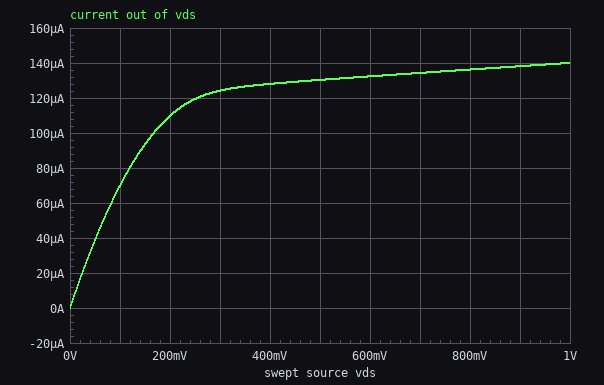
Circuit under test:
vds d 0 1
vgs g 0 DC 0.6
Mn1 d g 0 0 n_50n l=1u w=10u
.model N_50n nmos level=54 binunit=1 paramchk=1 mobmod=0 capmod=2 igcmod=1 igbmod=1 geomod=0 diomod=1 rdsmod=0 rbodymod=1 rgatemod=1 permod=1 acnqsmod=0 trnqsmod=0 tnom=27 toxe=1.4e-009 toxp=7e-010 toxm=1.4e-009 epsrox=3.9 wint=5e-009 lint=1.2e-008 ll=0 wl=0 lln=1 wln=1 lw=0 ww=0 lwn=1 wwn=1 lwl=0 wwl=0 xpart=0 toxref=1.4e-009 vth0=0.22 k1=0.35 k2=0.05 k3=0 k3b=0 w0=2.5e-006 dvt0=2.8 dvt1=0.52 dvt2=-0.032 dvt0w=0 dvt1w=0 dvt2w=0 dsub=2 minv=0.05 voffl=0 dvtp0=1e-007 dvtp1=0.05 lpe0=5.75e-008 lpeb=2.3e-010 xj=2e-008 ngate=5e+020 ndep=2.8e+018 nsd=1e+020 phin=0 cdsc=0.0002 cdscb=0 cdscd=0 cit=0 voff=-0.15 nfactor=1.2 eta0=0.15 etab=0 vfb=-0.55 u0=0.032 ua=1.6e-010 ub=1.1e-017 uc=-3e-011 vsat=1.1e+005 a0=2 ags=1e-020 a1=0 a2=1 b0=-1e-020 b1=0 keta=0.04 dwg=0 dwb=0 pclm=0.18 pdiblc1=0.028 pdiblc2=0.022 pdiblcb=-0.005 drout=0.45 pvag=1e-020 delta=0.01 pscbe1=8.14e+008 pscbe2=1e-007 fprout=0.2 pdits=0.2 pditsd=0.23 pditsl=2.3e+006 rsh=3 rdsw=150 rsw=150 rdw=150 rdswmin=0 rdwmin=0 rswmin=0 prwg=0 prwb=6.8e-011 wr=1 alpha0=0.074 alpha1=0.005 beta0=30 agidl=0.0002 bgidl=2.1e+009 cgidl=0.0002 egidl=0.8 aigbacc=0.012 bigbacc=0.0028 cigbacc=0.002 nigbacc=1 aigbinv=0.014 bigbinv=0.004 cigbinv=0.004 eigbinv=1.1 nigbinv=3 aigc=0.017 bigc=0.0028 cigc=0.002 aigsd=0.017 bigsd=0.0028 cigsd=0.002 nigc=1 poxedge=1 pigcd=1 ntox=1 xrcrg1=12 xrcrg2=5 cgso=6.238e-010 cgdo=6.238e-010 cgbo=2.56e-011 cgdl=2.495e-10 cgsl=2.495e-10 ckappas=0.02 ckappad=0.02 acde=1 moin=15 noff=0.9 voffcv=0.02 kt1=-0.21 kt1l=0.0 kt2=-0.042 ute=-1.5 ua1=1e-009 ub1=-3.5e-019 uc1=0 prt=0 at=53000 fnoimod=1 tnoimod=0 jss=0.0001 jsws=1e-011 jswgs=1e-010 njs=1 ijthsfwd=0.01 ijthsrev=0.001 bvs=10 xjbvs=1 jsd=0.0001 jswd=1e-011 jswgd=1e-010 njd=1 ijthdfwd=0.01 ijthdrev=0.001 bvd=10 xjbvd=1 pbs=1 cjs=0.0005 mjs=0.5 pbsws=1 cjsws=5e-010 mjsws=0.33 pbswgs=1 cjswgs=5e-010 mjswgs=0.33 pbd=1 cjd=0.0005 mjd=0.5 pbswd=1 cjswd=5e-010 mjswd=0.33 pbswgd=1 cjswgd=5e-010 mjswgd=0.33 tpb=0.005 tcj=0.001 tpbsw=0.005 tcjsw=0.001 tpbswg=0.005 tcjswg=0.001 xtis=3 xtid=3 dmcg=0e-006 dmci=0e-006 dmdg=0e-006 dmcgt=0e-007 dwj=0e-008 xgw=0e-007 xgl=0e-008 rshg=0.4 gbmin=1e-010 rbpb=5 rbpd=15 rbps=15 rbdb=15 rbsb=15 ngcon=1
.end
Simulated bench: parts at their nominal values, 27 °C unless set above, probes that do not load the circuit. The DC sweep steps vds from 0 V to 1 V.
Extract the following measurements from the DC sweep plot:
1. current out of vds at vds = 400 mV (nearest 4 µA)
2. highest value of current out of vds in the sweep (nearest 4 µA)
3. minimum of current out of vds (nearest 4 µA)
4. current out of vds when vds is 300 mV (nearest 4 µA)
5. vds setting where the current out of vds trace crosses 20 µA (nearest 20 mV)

128 µA
140 µA
0 A
124 µA
20 mV
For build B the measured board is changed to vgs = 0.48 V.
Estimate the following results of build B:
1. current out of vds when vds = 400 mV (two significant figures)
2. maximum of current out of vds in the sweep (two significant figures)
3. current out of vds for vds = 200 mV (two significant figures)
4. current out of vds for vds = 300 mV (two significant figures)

77 µA
85 µA
71 µA
75 µA
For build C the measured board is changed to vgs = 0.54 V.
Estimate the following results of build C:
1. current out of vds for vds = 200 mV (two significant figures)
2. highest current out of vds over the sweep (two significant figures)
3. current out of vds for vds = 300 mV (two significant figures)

92 µA
110 µA
100 µA
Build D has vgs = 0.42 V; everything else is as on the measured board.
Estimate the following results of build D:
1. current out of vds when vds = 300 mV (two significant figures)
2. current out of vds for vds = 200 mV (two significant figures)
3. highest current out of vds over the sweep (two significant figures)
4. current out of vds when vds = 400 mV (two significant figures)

51 µA
49 µA
59 µA
52 µA
